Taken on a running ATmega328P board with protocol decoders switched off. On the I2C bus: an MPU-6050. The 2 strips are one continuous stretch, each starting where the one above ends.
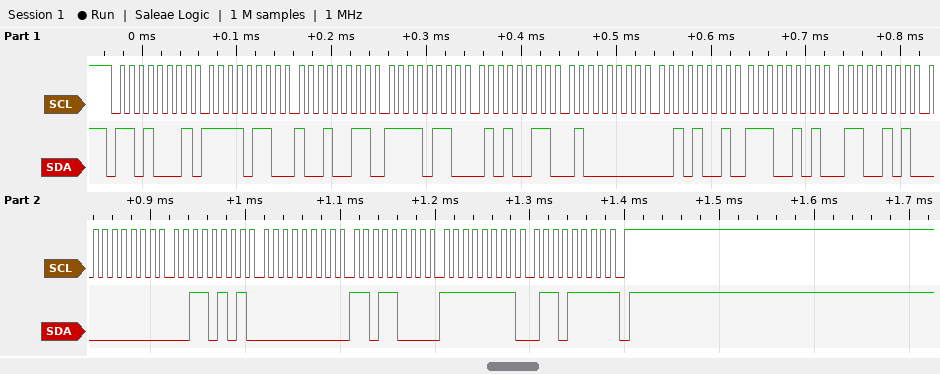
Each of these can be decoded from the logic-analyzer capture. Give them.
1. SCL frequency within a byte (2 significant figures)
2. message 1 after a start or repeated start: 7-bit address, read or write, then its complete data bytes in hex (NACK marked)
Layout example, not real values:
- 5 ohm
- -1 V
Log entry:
- 100 kHz
- 0x68 read: F6 93 F6 53 40 29 E5 65 00 35 00 D8 FF 6F NACK
